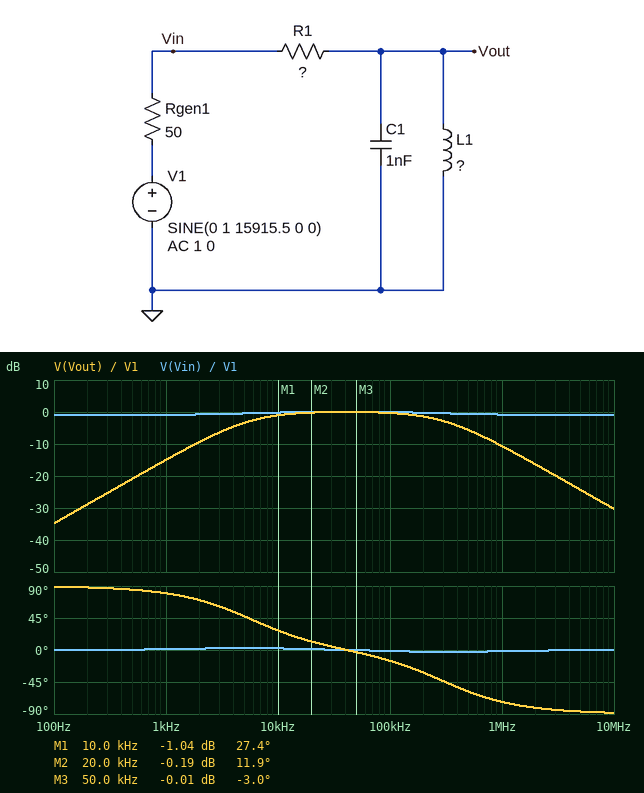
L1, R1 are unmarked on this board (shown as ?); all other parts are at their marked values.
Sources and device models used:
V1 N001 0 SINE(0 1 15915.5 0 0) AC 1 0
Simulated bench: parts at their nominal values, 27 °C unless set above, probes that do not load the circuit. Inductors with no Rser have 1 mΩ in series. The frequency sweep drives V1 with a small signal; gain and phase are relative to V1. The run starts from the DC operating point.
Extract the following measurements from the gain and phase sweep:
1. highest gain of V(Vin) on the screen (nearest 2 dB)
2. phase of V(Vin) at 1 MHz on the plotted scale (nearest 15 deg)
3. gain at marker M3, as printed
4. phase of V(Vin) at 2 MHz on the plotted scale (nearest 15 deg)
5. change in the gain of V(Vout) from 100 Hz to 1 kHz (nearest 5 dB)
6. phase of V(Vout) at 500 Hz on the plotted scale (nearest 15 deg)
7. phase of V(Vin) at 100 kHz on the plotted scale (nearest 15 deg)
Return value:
0 dB
0 deg
-0.01 dB
0 deg
20 dB
90 deg
0 deg
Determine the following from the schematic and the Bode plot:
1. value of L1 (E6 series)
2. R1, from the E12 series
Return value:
15 mH
470 Ω
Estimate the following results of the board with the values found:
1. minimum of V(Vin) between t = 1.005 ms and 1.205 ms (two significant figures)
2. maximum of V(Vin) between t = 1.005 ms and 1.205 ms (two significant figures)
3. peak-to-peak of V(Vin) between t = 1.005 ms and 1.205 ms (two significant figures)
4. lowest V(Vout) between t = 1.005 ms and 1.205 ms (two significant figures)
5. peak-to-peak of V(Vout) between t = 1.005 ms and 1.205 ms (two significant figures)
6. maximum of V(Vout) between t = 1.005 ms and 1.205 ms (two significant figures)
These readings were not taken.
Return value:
-990 mV
990 mV
2.0 V
-960 mV
1.9 V
960 mV
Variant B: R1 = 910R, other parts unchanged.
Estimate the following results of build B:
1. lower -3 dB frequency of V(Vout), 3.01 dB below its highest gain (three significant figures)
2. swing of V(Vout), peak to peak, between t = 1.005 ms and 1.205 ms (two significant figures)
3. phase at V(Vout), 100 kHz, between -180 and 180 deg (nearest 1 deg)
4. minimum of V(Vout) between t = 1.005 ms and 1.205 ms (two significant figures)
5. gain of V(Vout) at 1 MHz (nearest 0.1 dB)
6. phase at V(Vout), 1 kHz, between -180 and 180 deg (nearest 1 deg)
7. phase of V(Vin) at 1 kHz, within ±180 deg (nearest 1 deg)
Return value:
9.63 kHz
1.8 V
-27 deg
-880 mV
-15.7 dB
84 deg
0 deg
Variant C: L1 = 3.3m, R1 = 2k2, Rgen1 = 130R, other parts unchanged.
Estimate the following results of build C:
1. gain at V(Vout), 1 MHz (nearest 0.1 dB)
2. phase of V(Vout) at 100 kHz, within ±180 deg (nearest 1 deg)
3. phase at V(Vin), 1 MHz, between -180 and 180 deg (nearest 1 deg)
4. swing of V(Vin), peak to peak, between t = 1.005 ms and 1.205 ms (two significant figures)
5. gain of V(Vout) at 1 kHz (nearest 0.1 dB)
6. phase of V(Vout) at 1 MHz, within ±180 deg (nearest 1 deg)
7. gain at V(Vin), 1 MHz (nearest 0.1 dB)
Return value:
-23.3 dB
-19 deg
0 deg
1.9 V
-41.0 dB
-86 deg
-0.5 dB
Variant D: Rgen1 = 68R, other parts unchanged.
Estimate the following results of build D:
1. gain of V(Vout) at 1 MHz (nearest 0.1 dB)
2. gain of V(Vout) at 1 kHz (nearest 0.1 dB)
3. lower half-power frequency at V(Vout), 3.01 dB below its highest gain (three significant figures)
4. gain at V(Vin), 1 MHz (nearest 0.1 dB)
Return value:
-10.9 dB
-15.3 dB
5.60 kHz
-1.1 dB
